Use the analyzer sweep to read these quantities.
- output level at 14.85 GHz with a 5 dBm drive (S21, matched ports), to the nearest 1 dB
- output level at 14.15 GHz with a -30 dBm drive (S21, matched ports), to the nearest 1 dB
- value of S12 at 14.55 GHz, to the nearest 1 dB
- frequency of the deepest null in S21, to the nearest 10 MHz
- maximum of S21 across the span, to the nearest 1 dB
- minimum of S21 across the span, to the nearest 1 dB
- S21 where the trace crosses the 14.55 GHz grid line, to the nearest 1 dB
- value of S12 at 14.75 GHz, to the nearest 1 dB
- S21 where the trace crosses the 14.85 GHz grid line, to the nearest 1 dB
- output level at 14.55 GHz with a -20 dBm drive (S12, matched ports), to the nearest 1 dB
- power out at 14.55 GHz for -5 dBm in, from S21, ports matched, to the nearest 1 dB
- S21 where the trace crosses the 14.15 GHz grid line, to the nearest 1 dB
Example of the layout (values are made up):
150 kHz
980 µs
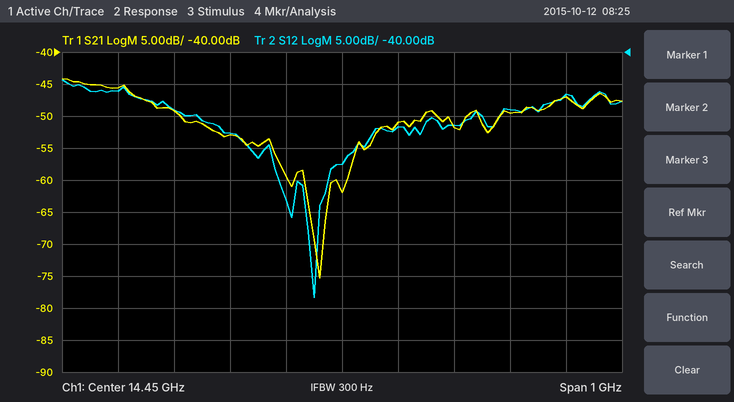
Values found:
-42 dBm
-79 dBm
-52 dB
14.41 GHz
-44 dB
-75 dB
-51 dB
-49 dB
-47 dB
-72 dBm
-56 dBm
-49 dB
